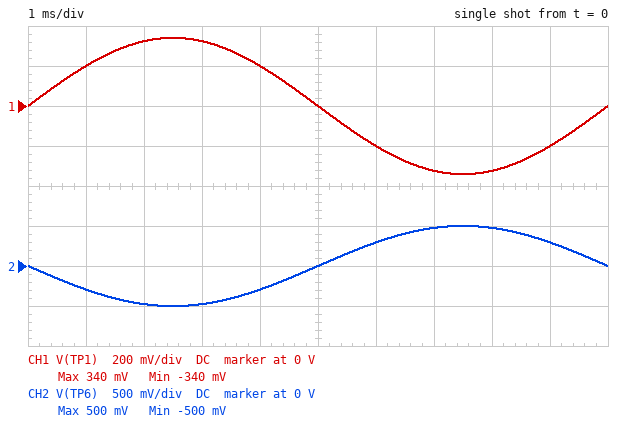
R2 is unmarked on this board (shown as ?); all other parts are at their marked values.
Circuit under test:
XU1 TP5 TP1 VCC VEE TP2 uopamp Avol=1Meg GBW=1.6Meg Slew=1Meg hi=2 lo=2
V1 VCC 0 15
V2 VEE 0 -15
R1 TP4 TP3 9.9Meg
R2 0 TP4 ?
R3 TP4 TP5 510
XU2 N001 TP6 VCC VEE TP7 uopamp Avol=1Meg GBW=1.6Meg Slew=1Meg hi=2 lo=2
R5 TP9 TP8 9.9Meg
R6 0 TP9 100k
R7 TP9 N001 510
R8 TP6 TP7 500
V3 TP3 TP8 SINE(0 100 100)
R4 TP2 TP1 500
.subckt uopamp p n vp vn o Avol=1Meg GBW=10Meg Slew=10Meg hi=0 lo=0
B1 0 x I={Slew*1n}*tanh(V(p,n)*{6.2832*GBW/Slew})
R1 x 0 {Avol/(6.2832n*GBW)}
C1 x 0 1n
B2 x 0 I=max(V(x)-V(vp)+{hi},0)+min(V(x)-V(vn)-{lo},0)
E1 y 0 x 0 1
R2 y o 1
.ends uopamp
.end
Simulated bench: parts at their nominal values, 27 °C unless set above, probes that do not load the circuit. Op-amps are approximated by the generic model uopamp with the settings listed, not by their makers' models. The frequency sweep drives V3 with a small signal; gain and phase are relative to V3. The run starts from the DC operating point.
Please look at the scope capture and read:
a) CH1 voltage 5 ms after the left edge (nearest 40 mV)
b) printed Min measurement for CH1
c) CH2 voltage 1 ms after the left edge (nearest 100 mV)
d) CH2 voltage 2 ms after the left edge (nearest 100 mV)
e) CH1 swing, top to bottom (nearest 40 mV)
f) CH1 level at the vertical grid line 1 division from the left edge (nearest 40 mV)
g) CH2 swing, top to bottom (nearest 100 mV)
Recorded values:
0 V
-340 mV
-300 mV
-500 mV
680 mV
200 mV
1.0 V
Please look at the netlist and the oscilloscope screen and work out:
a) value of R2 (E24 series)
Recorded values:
68 kΩ
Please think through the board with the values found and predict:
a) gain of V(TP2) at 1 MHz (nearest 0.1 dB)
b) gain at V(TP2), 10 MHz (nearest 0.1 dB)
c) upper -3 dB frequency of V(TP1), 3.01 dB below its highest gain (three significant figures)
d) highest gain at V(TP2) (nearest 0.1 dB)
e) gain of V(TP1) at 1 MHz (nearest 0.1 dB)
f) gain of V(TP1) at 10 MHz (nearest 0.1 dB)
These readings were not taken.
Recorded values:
-50.8 dB
-65.4 dB
1.60 MHz
-49.4 dB
-50.8 dB
-65.4 dB
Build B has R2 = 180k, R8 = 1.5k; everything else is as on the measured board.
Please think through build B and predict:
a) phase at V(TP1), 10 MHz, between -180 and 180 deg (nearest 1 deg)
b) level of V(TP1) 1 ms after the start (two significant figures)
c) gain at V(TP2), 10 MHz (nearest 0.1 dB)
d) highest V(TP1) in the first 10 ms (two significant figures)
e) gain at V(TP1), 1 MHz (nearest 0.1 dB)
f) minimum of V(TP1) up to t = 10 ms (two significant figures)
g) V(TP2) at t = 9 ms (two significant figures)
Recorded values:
-81 deg
530 mV
-57.0 dB
900 mV
-42.4 dB
-900 mV
-530 mV
